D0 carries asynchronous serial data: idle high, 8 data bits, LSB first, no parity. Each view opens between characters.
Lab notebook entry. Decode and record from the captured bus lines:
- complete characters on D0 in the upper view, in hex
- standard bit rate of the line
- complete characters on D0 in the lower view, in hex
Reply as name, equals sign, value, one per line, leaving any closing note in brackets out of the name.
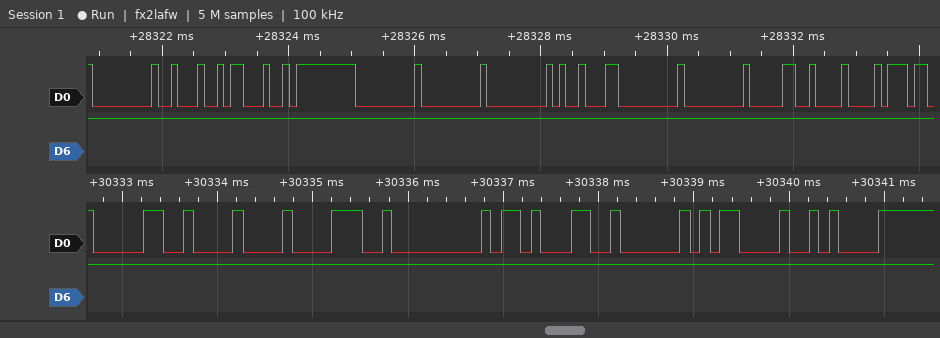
complete characters on D0 in the upper view, in hex = 00, 22, 23, FF, 00, 00, 00, 89, 00, 00, 30, 08
standard bit rate of the line = 9600 baud
complete characters on D0 in the lower view, in hex = 30, 08, 38, 00, 8B, 02, 0D, 0A
